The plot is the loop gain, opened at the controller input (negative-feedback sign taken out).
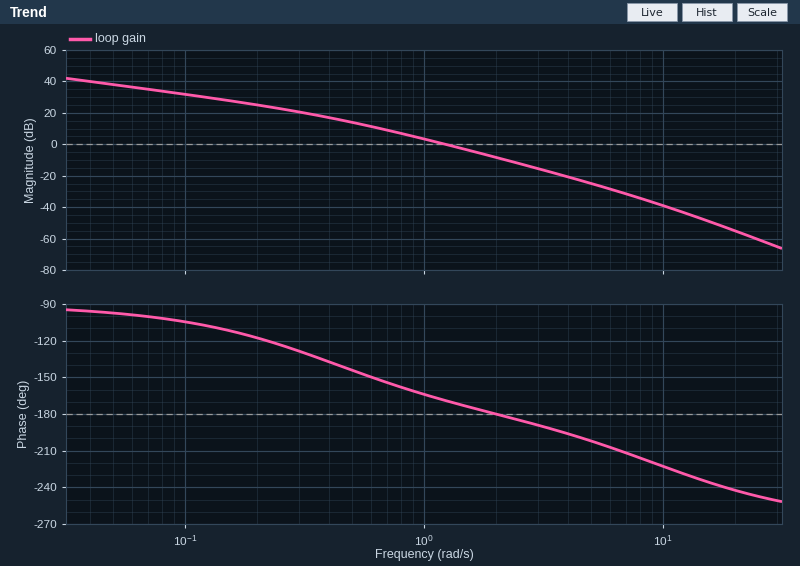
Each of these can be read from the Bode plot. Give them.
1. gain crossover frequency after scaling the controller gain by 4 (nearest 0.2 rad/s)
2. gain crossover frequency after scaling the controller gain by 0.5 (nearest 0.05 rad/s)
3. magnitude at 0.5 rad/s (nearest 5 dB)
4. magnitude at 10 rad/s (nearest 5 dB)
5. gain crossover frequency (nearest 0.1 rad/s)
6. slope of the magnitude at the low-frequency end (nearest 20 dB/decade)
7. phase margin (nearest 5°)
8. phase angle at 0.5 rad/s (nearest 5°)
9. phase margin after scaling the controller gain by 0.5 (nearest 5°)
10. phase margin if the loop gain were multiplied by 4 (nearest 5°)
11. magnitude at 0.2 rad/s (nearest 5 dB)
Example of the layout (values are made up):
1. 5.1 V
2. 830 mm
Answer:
1. 2.4 rad/s
2. 0.85 rad/s
3. 15 dB
4. -40 dB
5. 1.2 rad/s
6. -20 dB/decade
7. 10°
8. -145°
9. 20°
10. -5°
11. 25 dB
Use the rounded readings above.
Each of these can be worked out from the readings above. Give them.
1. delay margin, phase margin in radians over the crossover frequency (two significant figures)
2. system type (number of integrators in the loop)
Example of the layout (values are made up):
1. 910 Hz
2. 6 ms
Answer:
1. 0.15 s
2. 1
